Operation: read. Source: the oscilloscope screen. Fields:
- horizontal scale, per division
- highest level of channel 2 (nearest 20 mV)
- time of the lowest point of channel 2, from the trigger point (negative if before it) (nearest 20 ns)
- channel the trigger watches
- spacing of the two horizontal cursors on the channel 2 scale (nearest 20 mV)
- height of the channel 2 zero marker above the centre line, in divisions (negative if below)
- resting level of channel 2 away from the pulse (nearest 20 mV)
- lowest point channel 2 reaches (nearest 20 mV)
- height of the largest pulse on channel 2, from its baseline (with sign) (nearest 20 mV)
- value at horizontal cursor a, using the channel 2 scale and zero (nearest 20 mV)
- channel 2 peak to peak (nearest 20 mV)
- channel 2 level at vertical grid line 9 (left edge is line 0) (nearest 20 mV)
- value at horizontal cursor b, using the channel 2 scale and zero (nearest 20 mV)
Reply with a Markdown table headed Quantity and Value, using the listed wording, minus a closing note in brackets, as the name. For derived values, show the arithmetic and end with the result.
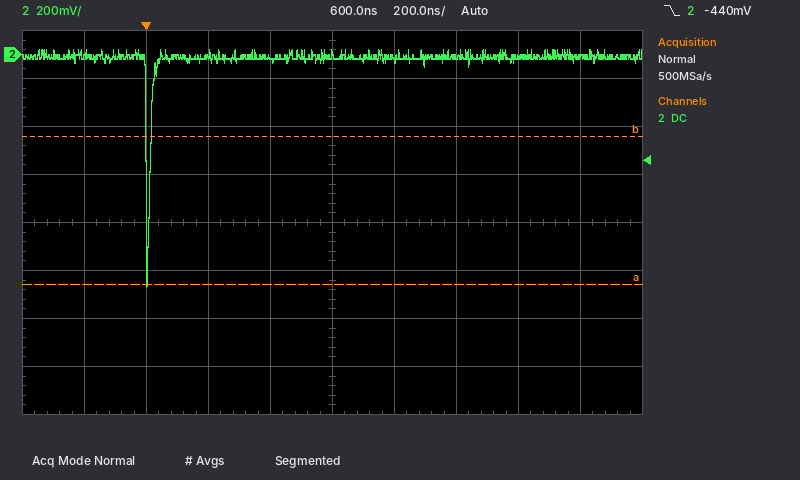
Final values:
| Quantity | Value |
|---|---|
| horizontal scale, per division | 200 ns |
| highest level of channel 2 | 20 mV |
| time of the lowest point of channel 2, from the trigger point (negative if before it) | 0 ns |
| channel the trigger watches | channel 2 |
| spacing of the two horizontal cursors on the channel 2 scale | 620 mV |
| height of the channel 2 zero marker above the centre line, in divisions | +3.5 div |
| resting level of channel 2 away from the pulse | 0 mV |
| lowest point channel 2 reaches | -960 mV |
| height of the largest pulse on channel 2, from its baseline (with sign) | -960 mV − (0 mV) = -960 mV |
| value at horizontal cursor a, using the channel 2 scale and zero | -960 mV |
| channel 2 peak to peak | 20 mV − (-960 mV) = 980 mV |
| channel 2 level at vertical grid line 9 (left edge is line 0) | 0 mV |
| value at horizontal cursor b, using the channel 2 scale and zero | -340 mV |
